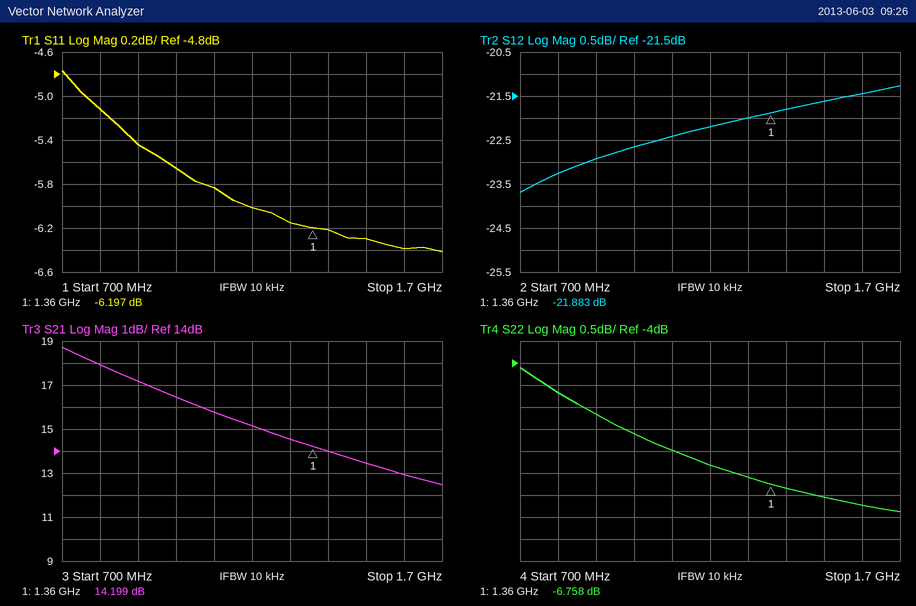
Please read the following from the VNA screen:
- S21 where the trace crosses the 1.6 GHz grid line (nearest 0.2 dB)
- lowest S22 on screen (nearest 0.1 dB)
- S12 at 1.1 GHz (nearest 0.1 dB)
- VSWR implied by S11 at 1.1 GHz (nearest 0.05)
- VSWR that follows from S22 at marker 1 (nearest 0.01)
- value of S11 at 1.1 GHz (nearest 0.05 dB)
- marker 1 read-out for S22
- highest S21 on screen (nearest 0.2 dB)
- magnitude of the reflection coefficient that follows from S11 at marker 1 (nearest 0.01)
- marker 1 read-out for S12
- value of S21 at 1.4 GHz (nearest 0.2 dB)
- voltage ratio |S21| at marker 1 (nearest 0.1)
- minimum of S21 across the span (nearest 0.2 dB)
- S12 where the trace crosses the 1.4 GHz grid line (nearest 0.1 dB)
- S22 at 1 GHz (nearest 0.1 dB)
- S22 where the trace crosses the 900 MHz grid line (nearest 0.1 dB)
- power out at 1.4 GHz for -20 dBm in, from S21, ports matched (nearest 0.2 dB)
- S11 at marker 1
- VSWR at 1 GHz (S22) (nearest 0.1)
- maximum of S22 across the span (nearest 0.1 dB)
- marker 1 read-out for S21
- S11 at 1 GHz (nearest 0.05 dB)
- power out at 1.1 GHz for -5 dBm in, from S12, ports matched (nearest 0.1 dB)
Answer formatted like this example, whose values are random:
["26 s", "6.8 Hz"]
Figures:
["13.0 dB", "-7.4 dB", "-22.4 dB", "3.10", "2.70", "-5.85 dB", "-6.758 dB", "18.8 dB", "0.49", "-21.883 dB", "14.0 dB", "5.1", "12.4 dB", "-21.8 dB", "-5.6 dB", "-5.2 dB", "-6.0 dBm", "-6.197 dB", "3.2", "-4.1 dB", "14.199 dB", "-5.65 dB", "-27.4 dBm"]
